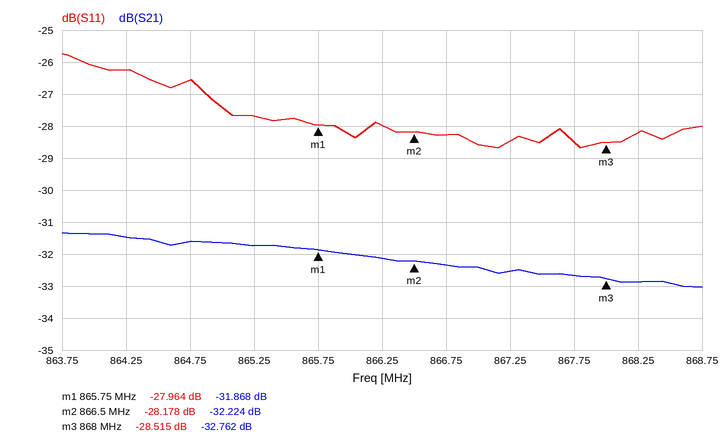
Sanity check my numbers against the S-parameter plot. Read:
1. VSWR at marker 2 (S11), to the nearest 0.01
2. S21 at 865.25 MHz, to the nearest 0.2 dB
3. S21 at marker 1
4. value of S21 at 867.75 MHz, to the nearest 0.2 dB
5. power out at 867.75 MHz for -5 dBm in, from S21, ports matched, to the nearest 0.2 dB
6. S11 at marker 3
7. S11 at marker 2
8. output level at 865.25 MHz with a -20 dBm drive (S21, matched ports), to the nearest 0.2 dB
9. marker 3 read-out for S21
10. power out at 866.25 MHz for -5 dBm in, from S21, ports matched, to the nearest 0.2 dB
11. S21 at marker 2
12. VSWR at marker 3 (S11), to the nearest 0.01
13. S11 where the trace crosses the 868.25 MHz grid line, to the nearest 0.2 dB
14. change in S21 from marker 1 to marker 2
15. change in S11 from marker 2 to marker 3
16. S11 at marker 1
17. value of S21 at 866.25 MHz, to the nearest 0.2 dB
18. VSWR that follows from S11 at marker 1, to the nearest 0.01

1.08
-31.8 dB
-31.868 dB
-32.6 dB
-37.6 dBm
-28.515 dB
-28.178 dB
-51.8 dBm
-32.762 dB
-37.2 dBm
-32.224 dB
1.08
-28.2 dB
-0.356 dB
-0.337 dB
-27.964 dB
-32.2 dB
1.08
